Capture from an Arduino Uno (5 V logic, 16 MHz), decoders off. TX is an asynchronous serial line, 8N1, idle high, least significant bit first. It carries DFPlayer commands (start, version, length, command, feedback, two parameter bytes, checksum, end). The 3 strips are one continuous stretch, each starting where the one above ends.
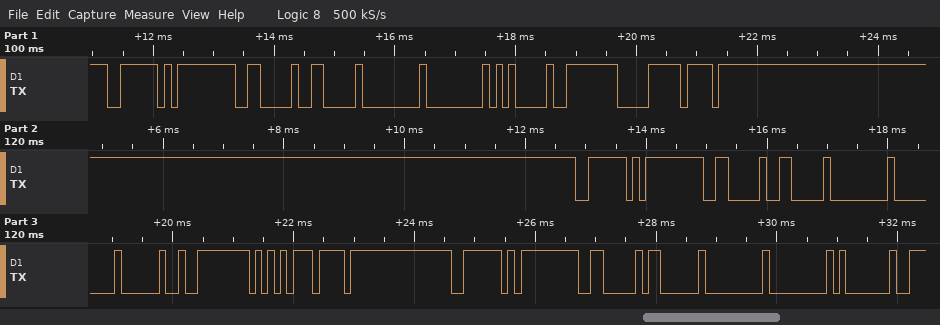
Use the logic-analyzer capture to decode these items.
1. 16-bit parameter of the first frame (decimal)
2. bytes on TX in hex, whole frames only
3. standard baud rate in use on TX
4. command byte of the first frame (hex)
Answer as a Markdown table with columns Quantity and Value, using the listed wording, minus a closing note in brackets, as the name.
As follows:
| Quantity | Value |
|---|---|
| 16-bit parameter of the first frame | 5 |
| bytes on TX in hex, whole frames only | 0x7E 0xFF 0x06 0x06 0x00 0x00 0x05 0xFE 0xF0 0xEF 0x7E 0xFF 0x06 0x06 0x00 0x00 0x20 0xFE 0xD5 0xEF 0x7E 0xFF 0x06 0x03 0x00 0x00 0x01 |
| standard baud rate in use on TX | 9600 baud |
| command byte of the first frame | 0x06 |
